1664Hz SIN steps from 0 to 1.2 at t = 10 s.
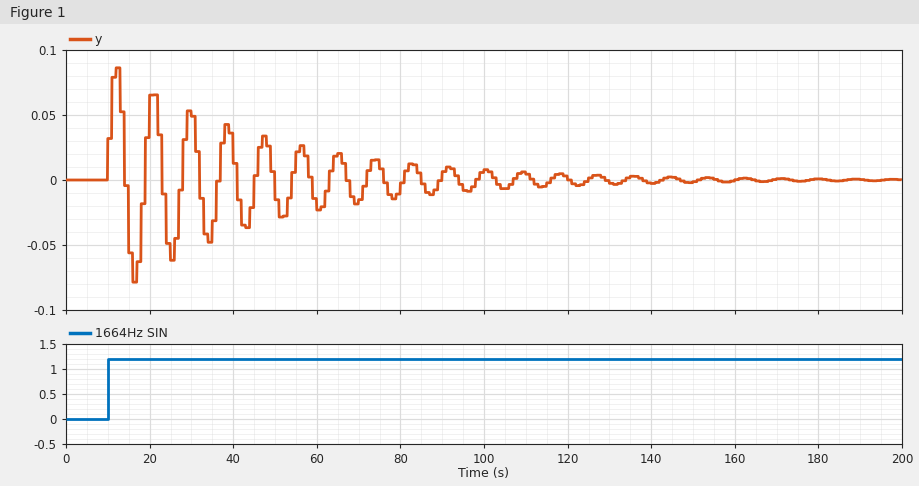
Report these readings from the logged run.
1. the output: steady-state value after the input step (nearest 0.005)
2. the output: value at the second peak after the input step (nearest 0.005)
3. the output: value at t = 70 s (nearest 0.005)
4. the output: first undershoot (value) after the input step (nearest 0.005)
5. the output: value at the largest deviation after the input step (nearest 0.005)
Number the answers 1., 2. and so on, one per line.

1. 0.000
2. 0.065
3. -0.015
4. -0.080
5. 0.085
